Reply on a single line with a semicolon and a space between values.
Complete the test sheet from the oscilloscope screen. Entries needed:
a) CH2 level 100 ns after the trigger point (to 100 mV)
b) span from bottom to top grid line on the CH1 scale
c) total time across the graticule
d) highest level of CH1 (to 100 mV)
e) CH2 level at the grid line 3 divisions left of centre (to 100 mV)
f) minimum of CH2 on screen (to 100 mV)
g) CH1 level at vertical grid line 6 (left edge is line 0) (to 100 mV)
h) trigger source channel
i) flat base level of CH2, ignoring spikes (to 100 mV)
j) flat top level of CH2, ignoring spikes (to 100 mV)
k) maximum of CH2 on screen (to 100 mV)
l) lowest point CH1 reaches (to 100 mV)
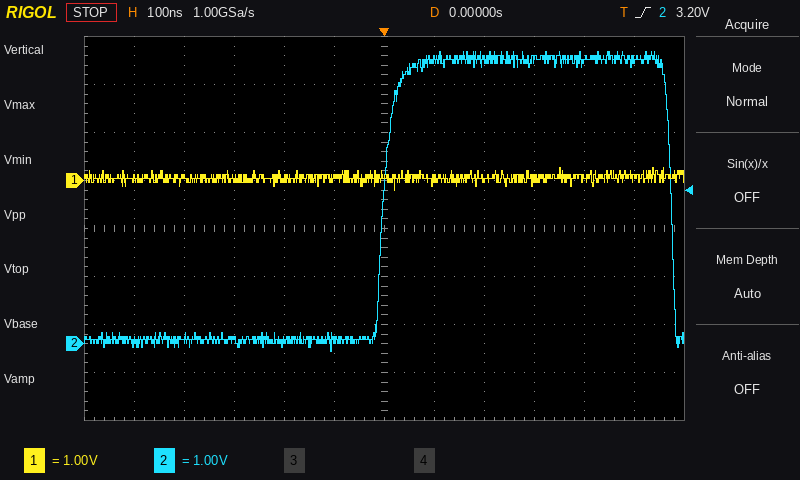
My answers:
5.9 V; 8 V; 1.2 µs; 300 mV; 100 mV; -200 mV; 100 mV; CH2; 100 mV; 5.9 V; 6.1 V; -200 mV
